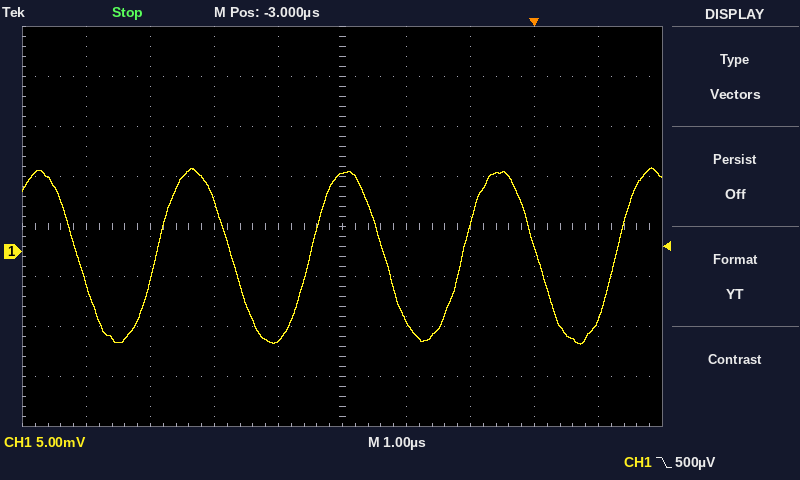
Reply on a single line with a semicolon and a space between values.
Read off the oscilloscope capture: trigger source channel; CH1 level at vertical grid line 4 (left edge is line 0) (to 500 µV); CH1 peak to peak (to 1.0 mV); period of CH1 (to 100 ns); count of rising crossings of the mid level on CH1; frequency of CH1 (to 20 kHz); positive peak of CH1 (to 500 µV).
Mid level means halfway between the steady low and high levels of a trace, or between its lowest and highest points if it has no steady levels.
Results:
CH1; -9.0 mV; 18.0 mV; 2.4 µs; 4; 420 kHz; 8.5 mV
